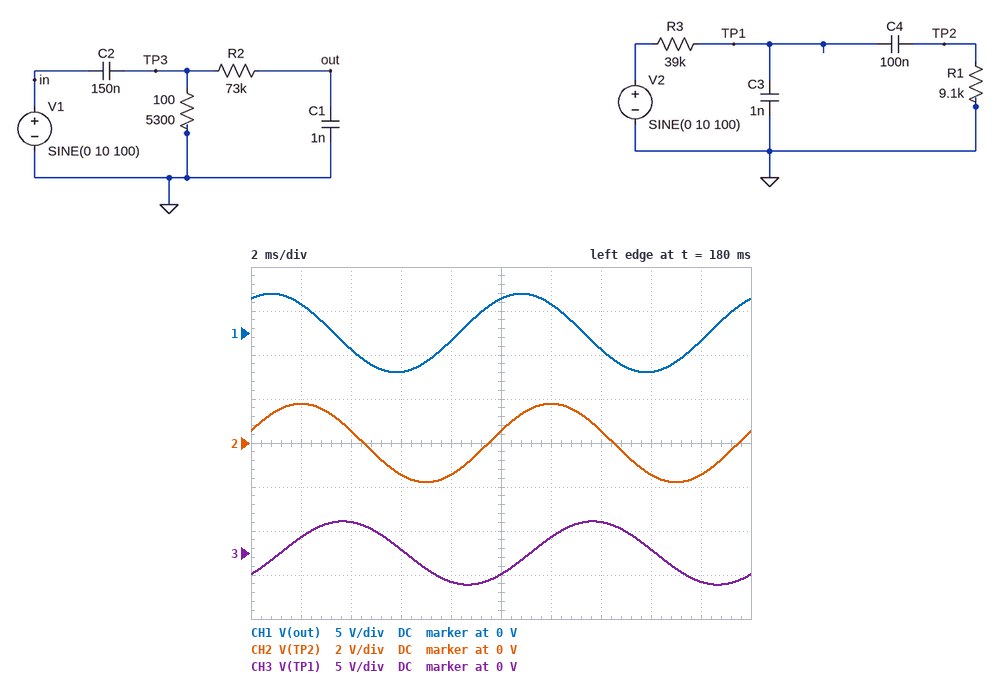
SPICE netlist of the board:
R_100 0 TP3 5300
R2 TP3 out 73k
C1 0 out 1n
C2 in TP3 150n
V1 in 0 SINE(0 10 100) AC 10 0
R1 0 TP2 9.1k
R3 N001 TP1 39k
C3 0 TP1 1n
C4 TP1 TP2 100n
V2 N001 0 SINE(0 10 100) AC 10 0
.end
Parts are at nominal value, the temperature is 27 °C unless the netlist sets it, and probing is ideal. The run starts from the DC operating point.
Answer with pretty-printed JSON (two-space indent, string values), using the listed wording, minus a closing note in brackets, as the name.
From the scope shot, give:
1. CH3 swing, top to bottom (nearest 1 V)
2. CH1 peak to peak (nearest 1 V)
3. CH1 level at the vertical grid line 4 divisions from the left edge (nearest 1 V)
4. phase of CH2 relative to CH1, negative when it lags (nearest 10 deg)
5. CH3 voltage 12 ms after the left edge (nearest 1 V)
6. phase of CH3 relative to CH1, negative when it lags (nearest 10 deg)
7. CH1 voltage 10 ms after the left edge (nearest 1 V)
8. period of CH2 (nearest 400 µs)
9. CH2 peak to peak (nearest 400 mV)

{
  "CH3 swing, top to bottom": "7 V",
  "CH1 peak to peak": "9 V",
  "CH1 level at the vertical grid line 4 divisions from the left edge": "-1 V",
  "phase of CH2 relative to CH1, negative when it lags": "-40 deg",
  "CH3 voltage 12 ms after the left edge": "2 V",
  "phase of CH3 relative to CH1, negative when it lags": "-100 deg",
  "CH1 voltage 10 ms after the left edge": "4 V",
  "period of CH2": "10.0 ms",
  "CH2 peak to peak": "3.6 V"
}
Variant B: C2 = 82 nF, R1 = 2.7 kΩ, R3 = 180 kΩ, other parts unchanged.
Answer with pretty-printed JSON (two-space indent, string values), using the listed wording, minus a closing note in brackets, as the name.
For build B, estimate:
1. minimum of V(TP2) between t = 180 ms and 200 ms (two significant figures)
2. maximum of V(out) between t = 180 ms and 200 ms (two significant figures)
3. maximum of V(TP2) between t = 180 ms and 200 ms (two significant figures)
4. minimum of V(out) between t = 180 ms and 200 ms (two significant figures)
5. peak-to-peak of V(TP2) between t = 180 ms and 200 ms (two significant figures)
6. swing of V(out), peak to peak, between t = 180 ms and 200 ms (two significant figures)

{
  "minimum of V(TP2) between t = 180 ms and 200 ms": "-150 mV",
  "maximum of V(out) between t = 180 ms and 200 ms": "2.6 V",
  "maximum of V(TP2) between t = 180 ms and 200 ms": "150 mV",
  "minimum of V(out) between t = 180 ms and 200 ms": "-2.6 V",
  "peak-to-peak of V(TP2) between t = 180 ms and 200 ms": "290 mV",
  "swing of V(out), peak to peak, between t = 180 ms and 200 ms": "5.3 V"
}
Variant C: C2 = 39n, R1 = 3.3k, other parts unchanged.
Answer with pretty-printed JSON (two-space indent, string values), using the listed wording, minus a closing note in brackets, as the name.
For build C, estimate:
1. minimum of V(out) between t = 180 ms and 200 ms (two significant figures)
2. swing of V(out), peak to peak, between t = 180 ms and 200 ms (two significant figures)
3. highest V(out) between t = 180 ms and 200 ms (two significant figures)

{
  "minimum of V(out) between t = 180 ms and 200 ms": "-1.3 V",
  "swing of V(out), peak to peak, between t = 180 ms and 200 ms": "2.6 V",
  "highest V(out) between t = 180 ms and 200 ms": "1.3 V"
}
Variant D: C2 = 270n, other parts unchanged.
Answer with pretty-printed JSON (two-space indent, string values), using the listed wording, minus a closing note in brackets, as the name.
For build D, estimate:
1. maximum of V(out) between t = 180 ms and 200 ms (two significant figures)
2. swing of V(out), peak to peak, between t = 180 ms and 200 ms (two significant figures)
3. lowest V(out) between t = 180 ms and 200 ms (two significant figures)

{
  "maximum of V(out) between t = 180 ms and 200 ms": "6.7 V",
  "swing of V(out), peak to peak, between t = 180 ms and 200 ms": "13 V",
  "lowest V(out) between t = 180 ms and 200 ms": "-6.7 V"
}
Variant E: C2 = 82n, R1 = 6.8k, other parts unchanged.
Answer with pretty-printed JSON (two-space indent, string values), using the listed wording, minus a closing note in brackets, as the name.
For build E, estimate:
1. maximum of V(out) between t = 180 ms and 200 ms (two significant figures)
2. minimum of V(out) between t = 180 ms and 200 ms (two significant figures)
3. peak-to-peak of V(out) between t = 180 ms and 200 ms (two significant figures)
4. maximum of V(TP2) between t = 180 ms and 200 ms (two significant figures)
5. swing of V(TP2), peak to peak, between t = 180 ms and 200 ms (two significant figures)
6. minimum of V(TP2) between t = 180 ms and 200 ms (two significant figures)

{
  "maximum of V(out) between t = 180 ms and 200 ms": "2.6 V",
  "minimum of V(out) between t = 180 ms and 200 ms": "-2.6 V",
  "peak-to-peak of V(out) between t = 180 ms and 200 ms": "5.3 V",
  "maximum of V(TP2) between t = 180 ms and 200 ms": "1.4 V",
  "swing of V(TP2), peak to peak, between t = 180 ms and 200 ms": "2.8 V",
  "minimum of V(TP2) between t = 180 ms and 200 ms": "-1.4 V"
}
